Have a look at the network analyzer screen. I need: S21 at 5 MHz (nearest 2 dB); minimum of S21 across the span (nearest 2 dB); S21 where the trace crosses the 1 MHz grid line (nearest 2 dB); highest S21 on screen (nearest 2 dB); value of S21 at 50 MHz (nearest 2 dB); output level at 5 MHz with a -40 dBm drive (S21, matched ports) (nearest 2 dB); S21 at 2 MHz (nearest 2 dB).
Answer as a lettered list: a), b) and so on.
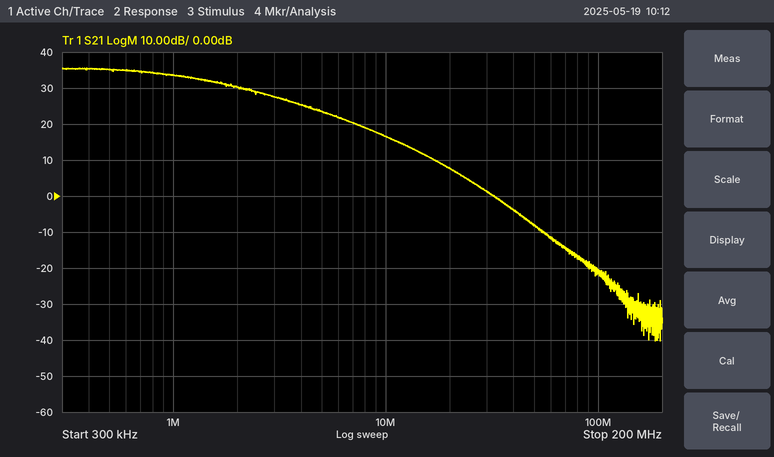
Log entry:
a) 24 dB
b) -40 dB
c) 34 dB
d) 36 dB
e) -8 dB
f) -16 dBm
g) 30 dB
